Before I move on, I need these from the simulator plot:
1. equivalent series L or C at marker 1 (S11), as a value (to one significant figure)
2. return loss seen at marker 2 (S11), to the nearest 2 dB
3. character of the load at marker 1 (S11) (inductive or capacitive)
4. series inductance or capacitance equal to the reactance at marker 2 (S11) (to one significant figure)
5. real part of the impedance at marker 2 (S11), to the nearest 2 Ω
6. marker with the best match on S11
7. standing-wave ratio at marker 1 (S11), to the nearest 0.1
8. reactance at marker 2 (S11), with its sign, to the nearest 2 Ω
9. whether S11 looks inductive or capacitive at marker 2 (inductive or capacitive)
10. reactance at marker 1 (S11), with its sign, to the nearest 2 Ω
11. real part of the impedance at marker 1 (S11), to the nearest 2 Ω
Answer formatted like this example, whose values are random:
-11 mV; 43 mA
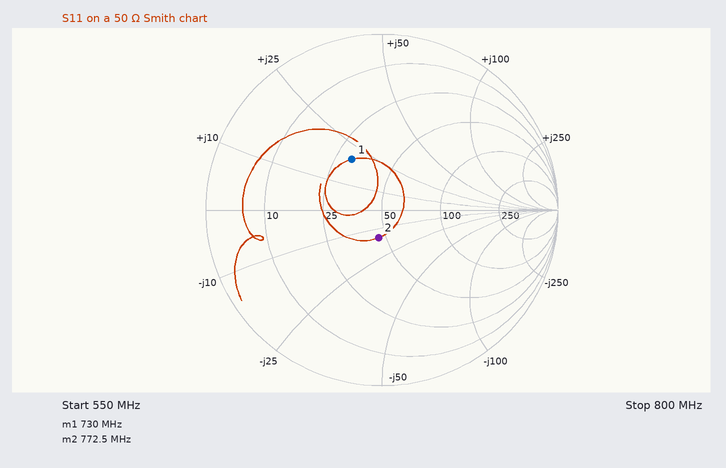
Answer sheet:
4 nH; 16 dB; inductive; 10 pF; 46 Ω; marker 2; 2.0; -14 Ω; capacitive; +20 Ω; 30 Ω
